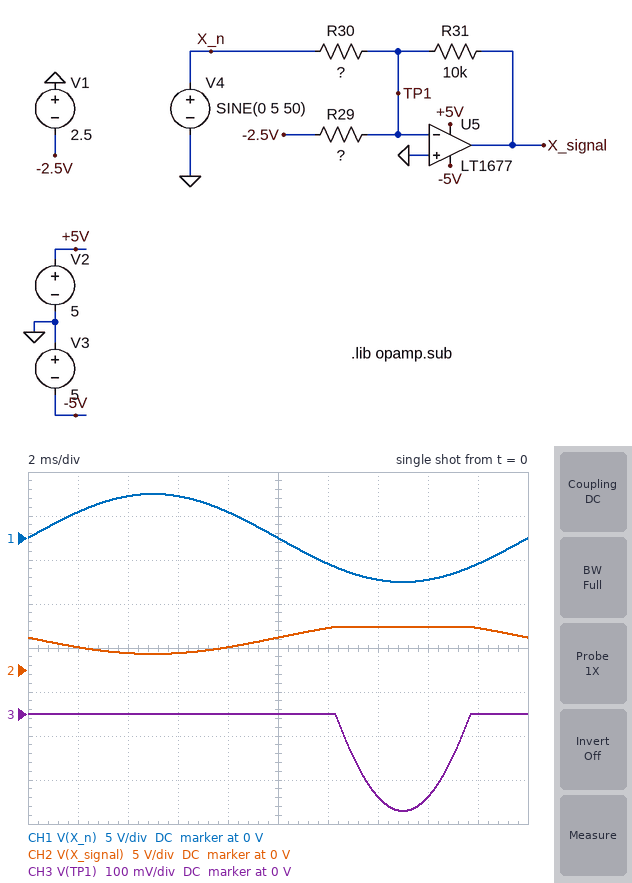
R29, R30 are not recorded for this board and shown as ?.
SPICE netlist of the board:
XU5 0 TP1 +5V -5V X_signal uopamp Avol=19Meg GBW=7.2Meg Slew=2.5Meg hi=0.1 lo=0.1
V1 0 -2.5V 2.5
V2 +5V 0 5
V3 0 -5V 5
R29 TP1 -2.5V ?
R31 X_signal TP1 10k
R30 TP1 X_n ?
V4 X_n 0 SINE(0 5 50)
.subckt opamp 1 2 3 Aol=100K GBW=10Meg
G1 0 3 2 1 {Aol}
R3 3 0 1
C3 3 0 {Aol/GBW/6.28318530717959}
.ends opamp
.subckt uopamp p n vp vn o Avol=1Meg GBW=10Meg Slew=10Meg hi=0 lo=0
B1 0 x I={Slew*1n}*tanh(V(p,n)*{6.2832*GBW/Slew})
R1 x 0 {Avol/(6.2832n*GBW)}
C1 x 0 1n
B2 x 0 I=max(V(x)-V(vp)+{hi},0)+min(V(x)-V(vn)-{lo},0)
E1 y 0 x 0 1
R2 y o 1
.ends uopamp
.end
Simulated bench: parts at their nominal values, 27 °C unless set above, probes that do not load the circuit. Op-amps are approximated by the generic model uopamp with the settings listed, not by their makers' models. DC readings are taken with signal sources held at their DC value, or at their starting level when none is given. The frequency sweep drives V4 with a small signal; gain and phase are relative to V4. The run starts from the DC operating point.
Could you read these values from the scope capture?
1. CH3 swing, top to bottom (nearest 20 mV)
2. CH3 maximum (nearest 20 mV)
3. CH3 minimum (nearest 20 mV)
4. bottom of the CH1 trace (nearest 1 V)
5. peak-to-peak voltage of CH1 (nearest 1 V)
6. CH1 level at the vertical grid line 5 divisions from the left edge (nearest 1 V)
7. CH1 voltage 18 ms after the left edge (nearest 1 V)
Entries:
220 mV
0 V
-220 mV
-5 V
10 V
0 V
-3 V
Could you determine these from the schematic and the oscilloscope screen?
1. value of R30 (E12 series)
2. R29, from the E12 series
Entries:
27 kΩ
6.8 kΩ
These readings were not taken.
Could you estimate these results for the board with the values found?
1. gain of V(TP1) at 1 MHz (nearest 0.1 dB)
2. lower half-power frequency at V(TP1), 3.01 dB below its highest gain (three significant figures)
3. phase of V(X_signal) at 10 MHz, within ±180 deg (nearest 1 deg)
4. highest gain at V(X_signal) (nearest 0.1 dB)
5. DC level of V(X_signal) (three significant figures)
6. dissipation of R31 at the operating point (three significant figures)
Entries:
-26.4 dB
2.53 MHz
104 deg
-8.6 dB
3.68 V
1.35 mW
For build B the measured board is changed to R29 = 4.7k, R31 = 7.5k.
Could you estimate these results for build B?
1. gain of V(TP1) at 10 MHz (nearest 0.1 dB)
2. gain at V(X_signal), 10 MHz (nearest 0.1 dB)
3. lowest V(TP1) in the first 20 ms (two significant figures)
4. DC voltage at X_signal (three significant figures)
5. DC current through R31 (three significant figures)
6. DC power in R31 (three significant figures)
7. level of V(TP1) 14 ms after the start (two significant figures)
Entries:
-20.6 dB
-23.4 dB
-170 mV
3.99 V
532 µA
2.12 mW
-140 mV
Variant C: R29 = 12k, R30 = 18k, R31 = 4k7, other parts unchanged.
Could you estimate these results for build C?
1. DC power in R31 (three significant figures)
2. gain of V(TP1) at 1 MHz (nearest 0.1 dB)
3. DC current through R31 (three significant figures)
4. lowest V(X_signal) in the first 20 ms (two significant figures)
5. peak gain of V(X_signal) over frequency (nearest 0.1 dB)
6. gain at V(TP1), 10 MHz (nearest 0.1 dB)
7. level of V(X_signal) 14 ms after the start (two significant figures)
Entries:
204 µW
-29.0 dB
208 µA
-330 mV
-11.7 dB
-16.8 dB
2.2 V
